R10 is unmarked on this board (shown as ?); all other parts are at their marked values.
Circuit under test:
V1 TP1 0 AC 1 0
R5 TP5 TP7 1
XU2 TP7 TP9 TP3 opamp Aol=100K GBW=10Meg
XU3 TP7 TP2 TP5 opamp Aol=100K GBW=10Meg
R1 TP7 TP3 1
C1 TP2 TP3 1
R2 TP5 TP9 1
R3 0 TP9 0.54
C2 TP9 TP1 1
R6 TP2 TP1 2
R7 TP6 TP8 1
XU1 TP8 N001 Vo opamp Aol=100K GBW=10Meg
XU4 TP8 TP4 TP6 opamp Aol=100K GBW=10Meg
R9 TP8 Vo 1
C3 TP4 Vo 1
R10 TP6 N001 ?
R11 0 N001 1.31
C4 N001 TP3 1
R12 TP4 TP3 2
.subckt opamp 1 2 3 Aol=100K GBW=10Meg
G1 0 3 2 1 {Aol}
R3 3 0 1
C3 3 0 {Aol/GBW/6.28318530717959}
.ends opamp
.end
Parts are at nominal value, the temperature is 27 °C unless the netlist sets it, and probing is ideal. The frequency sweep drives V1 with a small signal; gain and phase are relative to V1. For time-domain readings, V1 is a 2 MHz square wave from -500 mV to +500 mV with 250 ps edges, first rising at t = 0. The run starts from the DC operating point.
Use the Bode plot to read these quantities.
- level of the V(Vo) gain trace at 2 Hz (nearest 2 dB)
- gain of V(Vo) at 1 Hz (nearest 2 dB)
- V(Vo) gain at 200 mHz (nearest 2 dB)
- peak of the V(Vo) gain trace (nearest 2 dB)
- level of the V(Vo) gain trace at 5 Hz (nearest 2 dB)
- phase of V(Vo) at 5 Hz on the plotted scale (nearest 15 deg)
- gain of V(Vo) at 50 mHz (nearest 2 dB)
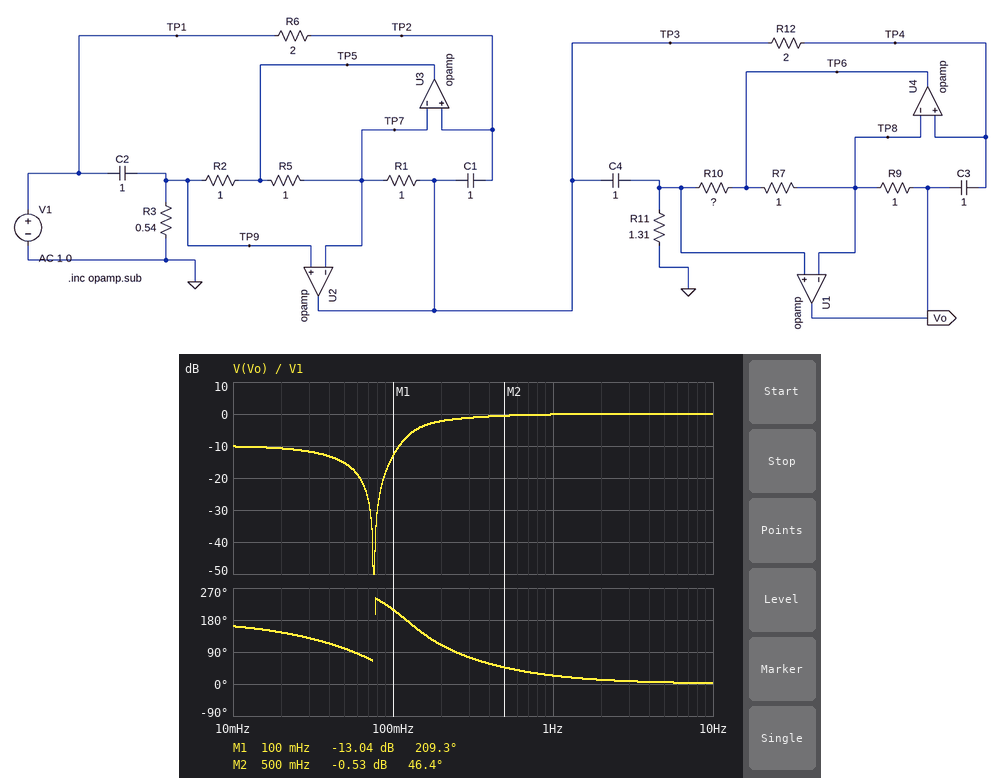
0 dB
0 dB
-2 dB
0 dB
0 dB
0 deg
-16 dB
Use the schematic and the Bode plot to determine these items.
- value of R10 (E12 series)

0.82 Ω
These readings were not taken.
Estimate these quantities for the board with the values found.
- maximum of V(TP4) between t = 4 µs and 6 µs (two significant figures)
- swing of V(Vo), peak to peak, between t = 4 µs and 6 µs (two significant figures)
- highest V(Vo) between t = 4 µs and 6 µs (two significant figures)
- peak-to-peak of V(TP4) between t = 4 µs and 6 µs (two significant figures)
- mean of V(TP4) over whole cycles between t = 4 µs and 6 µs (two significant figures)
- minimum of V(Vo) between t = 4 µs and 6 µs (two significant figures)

1.8 V
1.8 V
1.6 V
1.8 V
930 mV
-260 mV
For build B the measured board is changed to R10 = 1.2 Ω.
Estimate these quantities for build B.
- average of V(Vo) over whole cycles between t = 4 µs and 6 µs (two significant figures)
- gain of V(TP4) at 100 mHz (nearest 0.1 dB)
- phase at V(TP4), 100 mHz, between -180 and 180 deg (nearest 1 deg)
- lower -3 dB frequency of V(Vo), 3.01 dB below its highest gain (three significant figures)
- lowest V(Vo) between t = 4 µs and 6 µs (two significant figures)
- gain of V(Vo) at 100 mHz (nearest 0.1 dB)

540 mV
-29.9 dB
8 deg
141 mHz
-380 mV
-5.6 dB
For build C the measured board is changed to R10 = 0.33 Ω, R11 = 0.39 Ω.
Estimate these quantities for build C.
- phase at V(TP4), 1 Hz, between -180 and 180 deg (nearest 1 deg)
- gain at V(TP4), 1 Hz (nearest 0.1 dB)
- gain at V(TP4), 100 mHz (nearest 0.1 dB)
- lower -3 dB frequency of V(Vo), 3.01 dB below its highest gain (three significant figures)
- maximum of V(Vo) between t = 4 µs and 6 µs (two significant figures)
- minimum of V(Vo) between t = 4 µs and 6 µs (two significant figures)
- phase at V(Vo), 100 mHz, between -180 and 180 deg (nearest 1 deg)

40 deg
-0.9 dB
-7.9 dB
421 mHz
1.5 V
-350 mV
-140 deg
